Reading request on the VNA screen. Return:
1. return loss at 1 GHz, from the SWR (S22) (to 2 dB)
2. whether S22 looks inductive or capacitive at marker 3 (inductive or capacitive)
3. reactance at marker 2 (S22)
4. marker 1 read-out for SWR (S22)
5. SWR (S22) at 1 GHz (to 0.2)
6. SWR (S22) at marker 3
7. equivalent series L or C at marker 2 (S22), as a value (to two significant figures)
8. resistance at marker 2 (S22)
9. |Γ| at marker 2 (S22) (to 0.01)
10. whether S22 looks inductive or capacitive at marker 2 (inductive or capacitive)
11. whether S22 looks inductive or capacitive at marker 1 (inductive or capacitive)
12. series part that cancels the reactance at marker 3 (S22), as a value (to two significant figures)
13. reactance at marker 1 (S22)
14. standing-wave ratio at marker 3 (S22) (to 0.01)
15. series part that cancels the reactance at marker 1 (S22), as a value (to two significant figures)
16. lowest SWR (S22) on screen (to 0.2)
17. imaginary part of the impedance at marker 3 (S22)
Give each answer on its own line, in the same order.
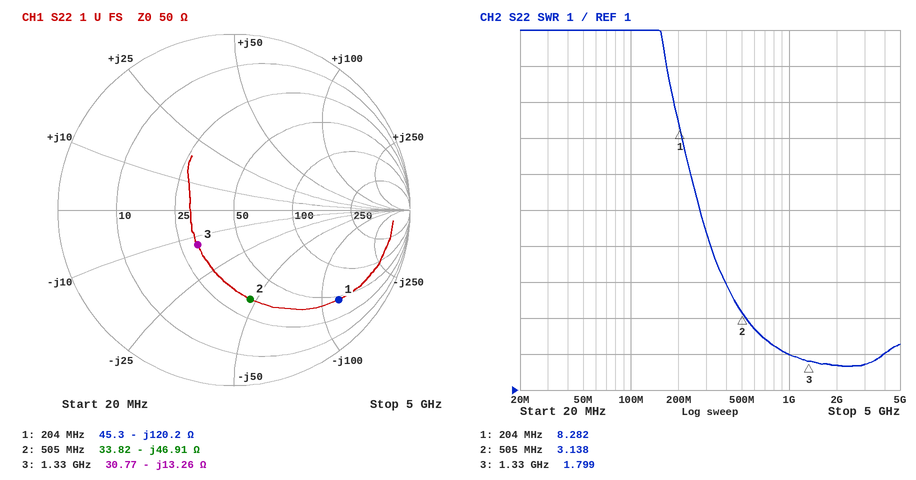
10 dB
capacitive
-46.91 Ω
8.282
2.0
1.799
6.7 pF
33.82 Ω
0.52
capacitive
capacitive
1.6 nH
-120.2 Ω
1.80
94 nH
1.6
-13.26 Ω
